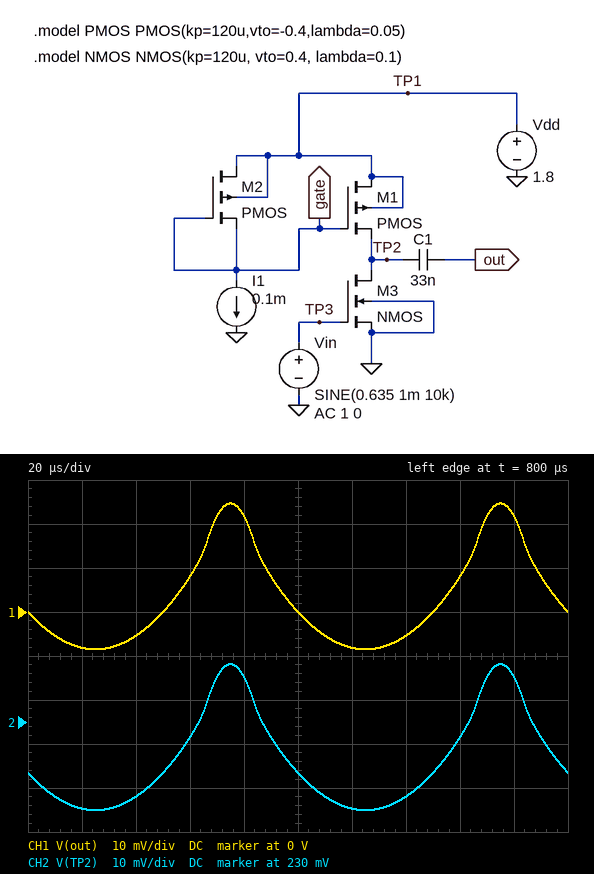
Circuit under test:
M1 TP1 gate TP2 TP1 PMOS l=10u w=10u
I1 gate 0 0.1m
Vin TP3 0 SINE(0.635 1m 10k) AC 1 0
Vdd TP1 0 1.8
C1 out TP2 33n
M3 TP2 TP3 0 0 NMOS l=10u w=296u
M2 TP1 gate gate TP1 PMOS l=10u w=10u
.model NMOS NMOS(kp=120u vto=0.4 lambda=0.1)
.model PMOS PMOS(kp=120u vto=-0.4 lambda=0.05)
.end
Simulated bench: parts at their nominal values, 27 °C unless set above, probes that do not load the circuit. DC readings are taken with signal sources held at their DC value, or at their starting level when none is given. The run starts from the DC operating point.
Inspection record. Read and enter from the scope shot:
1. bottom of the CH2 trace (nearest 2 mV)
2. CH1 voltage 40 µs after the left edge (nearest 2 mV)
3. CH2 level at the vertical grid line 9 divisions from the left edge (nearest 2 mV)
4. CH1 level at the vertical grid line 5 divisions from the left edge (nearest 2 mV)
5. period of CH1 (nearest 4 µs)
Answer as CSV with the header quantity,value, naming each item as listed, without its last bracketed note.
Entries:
quantity,value
bottom of the CH2 trace,210 mV
CH1 voltage 40 µs after the left edge,-6 mV
CH2 level at the vertical grid line 9 divisions from the left edge,240 mV
CH1 level at the vertical grid line 5 divisions from the left edge,0 V
period of CH1,100 µs
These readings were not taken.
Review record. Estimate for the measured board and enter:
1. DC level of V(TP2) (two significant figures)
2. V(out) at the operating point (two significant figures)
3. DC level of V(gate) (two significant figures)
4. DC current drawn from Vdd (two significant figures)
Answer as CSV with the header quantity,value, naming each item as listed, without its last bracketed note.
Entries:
quantity,value
DC level of V(TP2),220 mV
V(out) at the operating point,220 mV
DC level of V(gate),160 mV
DC current drawn from Vdd,200 µA
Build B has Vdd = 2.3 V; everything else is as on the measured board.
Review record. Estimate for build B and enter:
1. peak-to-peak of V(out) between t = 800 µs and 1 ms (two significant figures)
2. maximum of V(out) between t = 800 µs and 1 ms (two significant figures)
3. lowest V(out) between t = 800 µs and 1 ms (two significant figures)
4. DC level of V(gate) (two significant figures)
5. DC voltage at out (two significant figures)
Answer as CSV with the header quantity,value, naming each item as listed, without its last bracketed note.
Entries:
quantity,value
peak-to-peak of V(out) between t = 800 µs and 1 ms,120 mV
maximum of V(out) between t = 800 µs and 1 ms,60 mV
lowest V(out) between t = 800 µs and 1 ms,-60 mV
DC level of V(gate),660 mV
DC voltage at out,340 mV
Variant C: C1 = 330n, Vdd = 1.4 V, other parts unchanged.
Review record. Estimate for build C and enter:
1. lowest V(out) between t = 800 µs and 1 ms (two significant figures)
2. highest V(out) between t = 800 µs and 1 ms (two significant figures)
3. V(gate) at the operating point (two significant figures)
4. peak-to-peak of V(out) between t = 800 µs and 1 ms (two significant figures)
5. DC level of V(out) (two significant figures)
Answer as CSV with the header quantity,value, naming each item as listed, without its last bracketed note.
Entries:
quantity,value
lowest V(out) between t = 800 µs and 1 ms,-4.6 mV
highest V(out) between t = 800 µs and 1 ms,5.5 mV
V(gate) at the operating point,-240 mV
peak-to-peak of V(out) between t = 800 µs and 1 ms,10 mV
DC level of V(out),200 mV
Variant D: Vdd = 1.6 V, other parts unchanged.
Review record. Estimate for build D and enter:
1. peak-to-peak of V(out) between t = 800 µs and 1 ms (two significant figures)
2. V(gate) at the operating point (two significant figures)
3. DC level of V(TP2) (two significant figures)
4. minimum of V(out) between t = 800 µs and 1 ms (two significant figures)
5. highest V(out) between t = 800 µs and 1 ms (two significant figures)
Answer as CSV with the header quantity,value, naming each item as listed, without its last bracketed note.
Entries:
quantity,value
peak-to-peak of V(out) between t = 800 µs and 1 ms,14 mV
V(gate) at the operating point,-41 mV
DC level of V(TP2),210 mV
minimum of V(out) between t = 800 µs and 1 ms,-6.0 mV
highest V(out) between t = 800 µs and 1 ms,8.2 mV
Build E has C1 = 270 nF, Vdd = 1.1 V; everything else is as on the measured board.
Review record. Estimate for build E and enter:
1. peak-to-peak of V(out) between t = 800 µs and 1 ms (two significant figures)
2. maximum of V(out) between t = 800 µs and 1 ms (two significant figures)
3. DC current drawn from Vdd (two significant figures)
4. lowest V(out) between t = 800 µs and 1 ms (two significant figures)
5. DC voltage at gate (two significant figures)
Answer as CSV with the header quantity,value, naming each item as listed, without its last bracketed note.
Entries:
quantity,value
peak-to-peak of V(out) between t = 800 µs and 1 ms,3.9 mV
maximum of V(out) between t = 800 µs and 1 ms,2.0 mV
DC current drawn from Vdd,190 µA
lowest V(out) between t = 800 µs and 1 ms,-1.9 mV
DC voltage at gate,-540 mV
